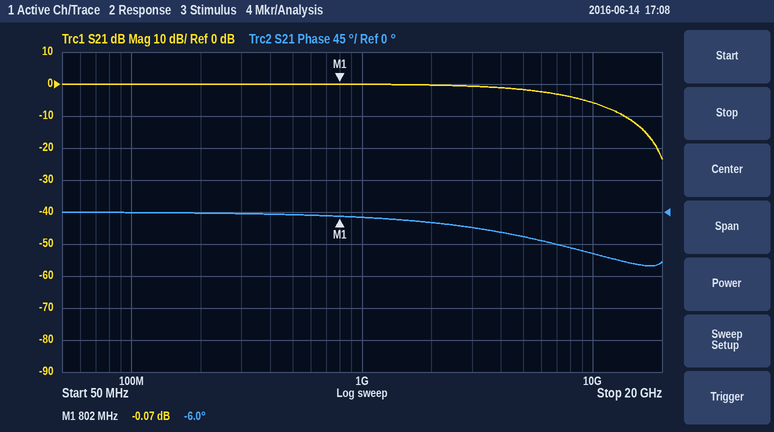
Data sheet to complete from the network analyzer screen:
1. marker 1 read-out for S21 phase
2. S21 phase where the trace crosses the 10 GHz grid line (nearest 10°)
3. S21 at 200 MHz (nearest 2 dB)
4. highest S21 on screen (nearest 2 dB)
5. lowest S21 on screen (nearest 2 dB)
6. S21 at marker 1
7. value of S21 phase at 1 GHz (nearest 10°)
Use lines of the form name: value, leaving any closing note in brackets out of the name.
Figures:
marker 1 read-out for S21 phase: -6.0°
S21 phase where the trace crosses the 10 GHz grid line: -60°
S21 at 200 MHz: 0 dB
highest S21 on screen: 0 dB
lowest S21 on screen: -24 dB
S21 at marker 1: -0.07 dB
value of S21 phase at 1 GHz: -10°
